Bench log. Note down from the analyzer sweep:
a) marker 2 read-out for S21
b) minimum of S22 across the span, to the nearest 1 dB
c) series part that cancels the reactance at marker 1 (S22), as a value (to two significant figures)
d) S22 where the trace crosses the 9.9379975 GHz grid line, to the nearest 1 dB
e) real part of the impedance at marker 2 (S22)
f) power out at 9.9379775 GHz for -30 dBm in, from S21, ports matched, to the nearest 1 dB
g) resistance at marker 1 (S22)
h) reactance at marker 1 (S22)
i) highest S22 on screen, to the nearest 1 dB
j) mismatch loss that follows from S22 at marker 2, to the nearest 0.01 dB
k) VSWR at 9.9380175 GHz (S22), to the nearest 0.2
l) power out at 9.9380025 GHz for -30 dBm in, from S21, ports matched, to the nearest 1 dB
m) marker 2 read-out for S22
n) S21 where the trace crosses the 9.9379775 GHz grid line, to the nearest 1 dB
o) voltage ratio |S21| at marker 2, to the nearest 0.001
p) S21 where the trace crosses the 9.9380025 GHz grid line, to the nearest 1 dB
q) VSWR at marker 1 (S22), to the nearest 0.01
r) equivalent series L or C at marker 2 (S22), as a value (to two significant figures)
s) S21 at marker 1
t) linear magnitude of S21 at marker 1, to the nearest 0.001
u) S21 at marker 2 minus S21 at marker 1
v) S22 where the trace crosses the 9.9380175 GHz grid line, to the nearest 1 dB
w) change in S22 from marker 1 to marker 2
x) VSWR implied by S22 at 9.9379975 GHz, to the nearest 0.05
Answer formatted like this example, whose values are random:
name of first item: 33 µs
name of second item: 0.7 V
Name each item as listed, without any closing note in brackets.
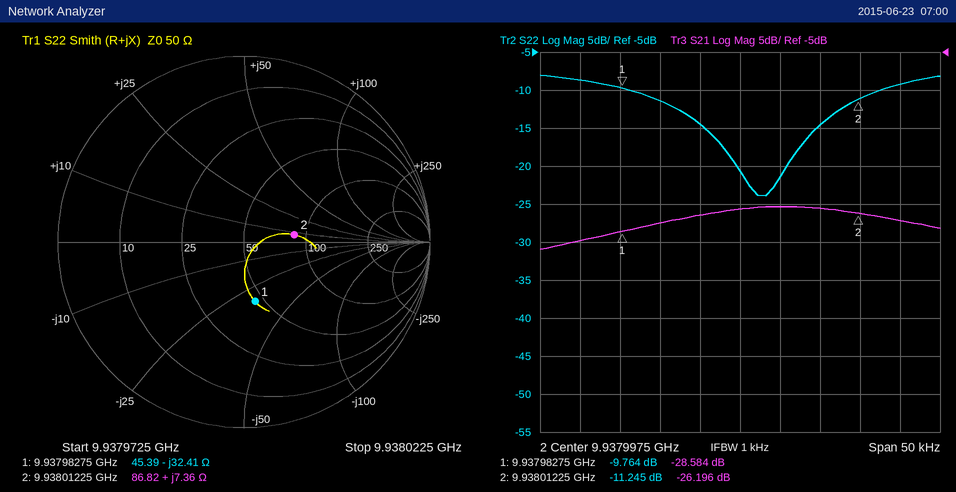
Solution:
marker 2 read-out for S21: -26.196 dB
minimum of S22 across the span, to the nearest 1 dB: -24 dB
series part that cancels the reactance at marker 1 (S22), as a value: 520 pH
S22 where the trace crosses the 9.9379975 GHz grid line, to the nearest 1 dB: -21 dB
real part of the impedance at marker 2: 86.82 Ω
power out at 9.9379775 GHz for -30 dBm in, from S21, ports matched, to the nearest 1 dB: -60 dBm
resistance at marker 1: 45.39 Ω
reactance at marker 1: -32.41 Ω
highest S22 on screen, to the nearest 1 dB: -8 dB
mismatch loss that follows from S22 at marker 2, to the nearest 0.01 dB: 0.34 dB
VSWR at 9.9380175 GHz (S22), to the nearest 0.2: 2.0
power out at 9.9380025 GHz for -30 dBm in, from S21, ports matched, to the nearest 1 dB: -55 dBm
marker 2 read-out for S22: -11.245 dB
S21 where the trace crosses the 9.9379775 GHz grid line, to the nearest 1 dB: -30 dB
voltage ratio |S21| at marker 2, to the nearest 0.001: 0.049
S21 where the trace crosses the 9.9380025 GHz grid line, to the nearest 1 dB: -25 dB
VSWR at marker 1 (S22), to the nearest 0.01: 1.96
equivalent series L or C at marker 2 (S22), as a value: 120 pH
S21 at marker 1: -28.584 dB
linear magnitude of S21 at marker 1, to the nearest 0.001: 0.037
S21 at marker 2 minus S21 at marker 1: 2.388 dB
S22 where the trace crosses the 9.9380175 GHz grid line, to the nearest 1 dB: -9 dB
change in S22 from marker 1 to marker 2: -1.481 dB
VSWR implied by S22 at 9.9379975 GHz, to the nearest 0.05: 1.20
